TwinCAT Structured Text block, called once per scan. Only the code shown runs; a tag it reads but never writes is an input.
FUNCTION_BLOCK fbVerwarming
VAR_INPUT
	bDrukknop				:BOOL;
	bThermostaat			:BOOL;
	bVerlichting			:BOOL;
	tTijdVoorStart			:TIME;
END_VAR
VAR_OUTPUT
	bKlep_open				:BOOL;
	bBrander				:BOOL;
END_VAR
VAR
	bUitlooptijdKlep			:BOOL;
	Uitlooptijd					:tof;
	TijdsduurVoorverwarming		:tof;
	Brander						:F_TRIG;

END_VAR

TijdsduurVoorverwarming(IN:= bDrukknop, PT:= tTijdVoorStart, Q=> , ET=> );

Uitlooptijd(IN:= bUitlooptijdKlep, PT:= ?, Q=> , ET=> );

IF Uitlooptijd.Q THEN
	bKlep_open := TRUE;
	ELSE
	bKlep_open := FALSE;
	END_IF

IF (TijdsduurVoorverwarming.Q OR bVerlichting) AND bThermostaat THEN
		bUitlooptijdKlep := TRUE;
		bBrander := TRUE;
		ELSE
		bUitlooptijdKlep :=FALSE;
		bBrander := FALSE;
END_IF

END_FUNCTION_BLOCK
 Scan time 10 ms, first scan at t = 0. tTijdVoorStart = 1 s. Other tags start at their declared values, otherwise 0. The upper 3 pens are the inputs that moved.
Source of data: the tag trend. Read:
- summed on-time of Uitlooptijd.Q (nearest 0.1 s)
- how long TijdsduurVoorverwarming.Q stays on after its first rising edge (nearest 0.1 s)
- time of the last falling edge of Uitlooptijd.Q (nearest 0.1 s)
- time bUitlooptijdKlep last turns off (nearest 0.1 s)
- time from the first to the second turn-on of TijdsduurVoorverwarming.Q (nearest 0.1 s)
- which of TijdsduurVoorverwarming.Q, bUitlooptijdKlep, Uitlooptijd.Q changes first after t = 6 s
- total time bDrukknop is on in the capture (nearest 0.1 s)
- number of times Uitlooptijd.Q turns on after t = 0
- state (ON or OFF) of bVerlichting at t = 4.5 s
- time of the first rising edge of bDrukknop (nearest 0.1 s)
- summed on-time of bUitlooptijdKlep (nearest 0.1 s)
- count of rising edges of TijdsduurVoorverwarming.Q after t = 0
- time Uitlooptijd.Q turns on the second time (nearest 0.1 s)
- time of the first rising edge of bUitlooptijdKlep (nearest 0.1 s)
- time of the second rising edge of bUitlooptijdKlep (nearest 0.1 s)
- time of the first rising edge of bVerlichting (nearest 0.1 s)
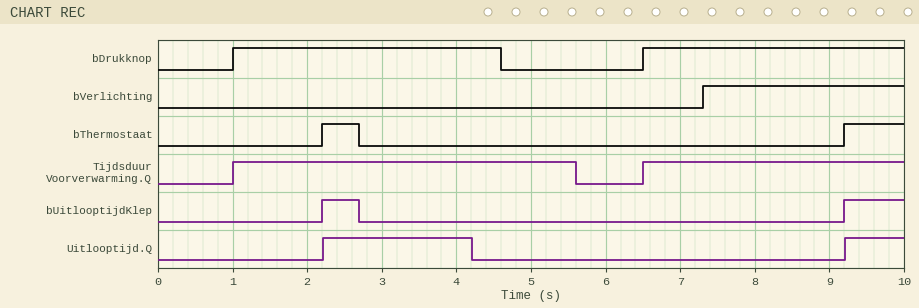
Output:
2.8 s
4.6 s
4.2 s
2.7 s
5.5 s
TijdsduurVoorverwarming.Q
7.1 s
2
OFF
1.0 s
1.3 s
2
9.2 s
2.2 s
9.2 s
7.3 s
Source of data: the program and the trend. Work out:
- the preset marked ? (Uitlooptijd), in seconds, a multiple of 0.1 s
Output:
1.5 s
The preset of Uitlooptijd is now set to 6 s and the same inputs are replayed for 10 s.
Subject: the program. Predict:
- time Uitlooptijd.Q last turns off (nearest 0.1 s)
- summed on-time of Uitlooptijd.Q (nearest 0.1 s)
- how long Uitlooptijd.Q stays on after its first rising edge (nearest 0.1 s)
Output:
8.7 s
7.3 s
6.5 s
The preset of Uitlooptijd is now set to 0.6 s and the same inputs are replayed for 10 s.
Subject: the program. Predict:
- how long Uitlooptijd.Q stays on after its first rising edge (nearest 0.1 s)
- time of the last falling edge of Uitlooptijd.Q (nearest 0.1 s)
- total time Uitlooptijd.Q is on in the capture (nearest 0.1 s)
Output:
1.1 s
3.3 s
1.9 s
